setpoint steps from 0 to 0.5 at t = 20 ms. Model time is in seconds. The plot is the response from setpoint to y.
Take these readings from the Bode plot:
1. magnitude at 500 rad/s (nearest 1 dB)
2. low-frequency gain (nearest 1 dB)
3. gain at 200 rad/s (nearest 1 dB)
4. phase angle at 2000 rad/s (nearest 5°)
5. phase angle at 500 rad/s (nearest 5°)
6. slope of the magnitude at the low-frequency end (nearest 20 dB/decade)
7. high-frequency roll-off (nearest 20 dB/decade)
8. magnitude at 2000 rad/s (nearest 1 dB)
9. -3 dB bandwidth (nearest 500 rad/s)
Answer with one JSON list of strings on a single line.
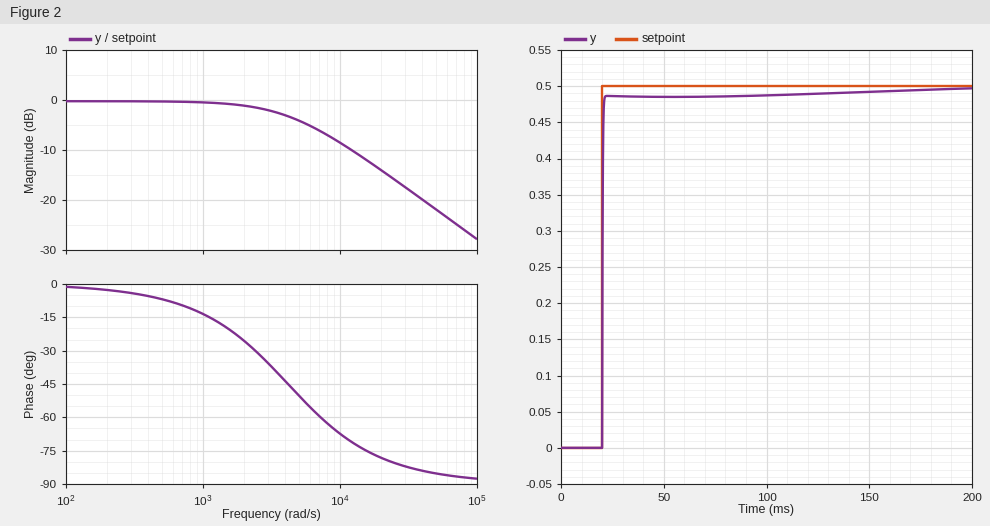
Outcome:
["0 dB", "0 dB", "0 dB", "-25°", "-5°", "0 dB/decade", "-20 dB/decade", "-1 dB", "4000 rad/s"]
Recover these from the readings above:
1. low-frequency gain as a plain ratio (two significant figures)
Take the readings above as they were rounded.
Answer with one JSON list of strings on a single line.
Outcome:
["1.0"]
